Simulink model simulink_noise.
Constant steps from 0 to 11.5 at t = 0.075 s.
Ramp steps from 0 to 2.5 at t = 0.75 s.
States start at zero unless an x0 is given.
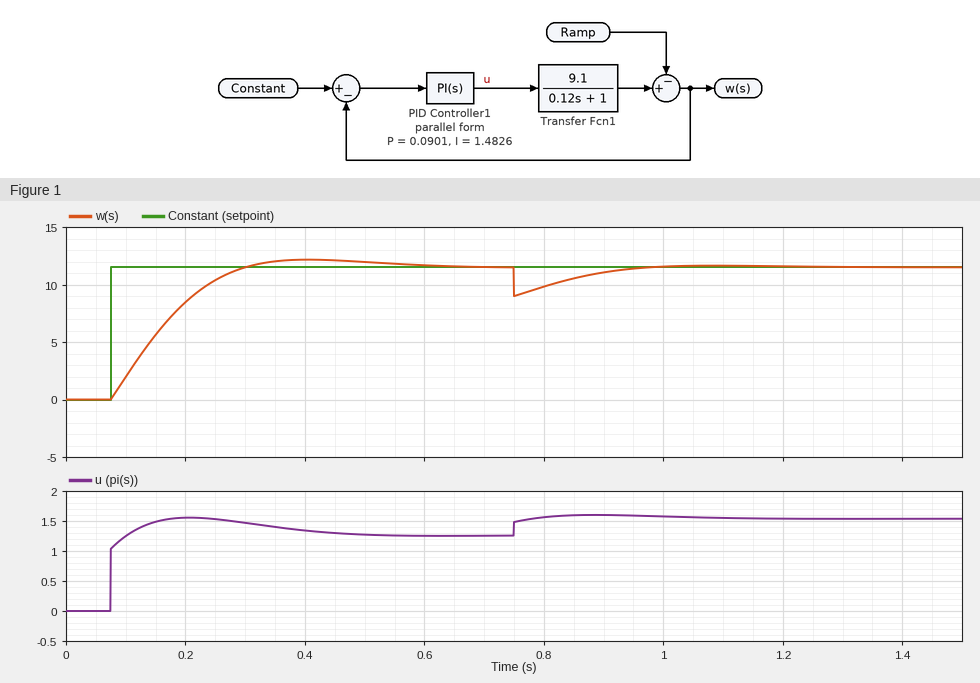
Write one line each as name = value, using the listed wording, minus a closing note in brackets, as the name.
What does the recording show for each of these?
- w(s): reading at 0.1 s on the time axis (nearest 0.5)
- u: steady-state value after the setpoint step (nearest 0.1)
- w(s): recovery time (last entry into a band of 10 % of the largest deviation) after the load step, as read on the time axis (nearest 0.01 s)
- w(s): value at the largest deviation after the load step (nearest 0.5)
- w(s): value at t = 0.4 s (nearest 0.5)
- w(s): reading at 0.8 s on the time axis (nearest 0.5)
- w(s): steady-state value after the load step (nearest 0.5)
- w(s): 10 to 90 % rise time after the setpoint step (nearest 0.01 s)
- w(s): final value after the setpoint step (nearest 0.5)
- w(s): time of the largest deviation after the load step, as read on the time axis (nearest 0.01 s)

w(s): reading at 0.1 s on the time axis = 2.0
u: steady-state value after the setpoint step = 1.3
w(s): recovery time (last entry into a band of 10 % of the largest deviation) after the load step, as read on the time axis = 0.93 s
w(s): value at the largest deviation after the load step = 9.0
w(s): value at t = 0.4 s = 12.0
w(s): reading at 0.8 s on the time axis = 10.0
w(s): steady-state value after the load step = 11.5
w(s): 10 to 90 % rise time after the setpoint step = 0.16 s
w(s): final value after the setpoint step = 11.5
w(s): time of the largest deviation after the load step, as read on the time axis = 0.75 s
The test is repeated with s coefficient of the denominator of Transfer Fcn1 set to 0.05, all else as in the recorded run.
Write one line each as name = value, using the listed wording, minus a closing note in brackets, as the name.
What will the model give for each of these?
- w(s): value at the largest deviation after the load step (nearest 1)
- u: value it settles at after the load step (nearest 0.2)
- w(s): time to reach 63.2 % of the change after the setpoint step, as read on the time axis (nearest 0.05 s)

w(s): value at the largest deviation after the load step = 9
u: value it settles at after the load step = 1.6
w(s): time to reach 63.2 % of the change after the setpoint step, as read on the time axis = 0.15 s
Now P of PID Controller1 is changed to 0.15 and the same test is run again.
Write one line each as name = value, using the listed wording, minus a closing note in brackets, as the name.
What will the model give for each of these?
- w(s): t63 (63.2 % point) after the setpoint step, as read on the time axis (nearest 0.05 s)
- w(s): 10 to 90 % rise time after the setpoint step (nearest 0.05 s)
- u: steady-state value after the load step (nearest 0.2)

w(s): t63 (63.2 % point) after the setpoint step, as read on the time axis = 0.15 s
w(s): 10 to 90 % rise time after the setpoint step = 0.15 s
u: steady-state value after the load step = 1.6
